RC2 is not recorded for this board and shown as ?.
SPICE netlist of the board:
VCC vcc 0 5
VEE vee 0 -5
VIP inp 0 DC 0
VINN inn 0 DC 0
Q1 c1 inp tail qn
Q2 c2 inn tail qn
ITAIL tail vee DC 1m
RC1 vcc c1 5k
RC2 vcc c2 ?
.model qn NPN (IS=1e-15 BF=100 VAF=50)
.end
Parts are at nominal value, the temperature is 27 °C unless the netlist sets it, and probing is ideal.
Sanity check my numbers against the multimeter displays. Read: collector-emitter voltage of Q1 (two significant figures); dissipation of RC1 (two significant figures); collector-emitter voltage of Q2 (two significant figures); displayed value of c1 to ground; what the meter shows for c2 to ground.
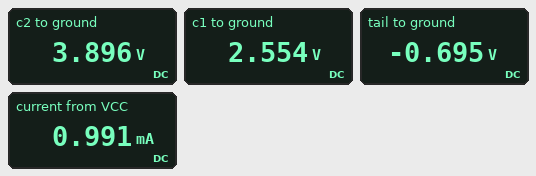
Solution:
3.2 V
1.2 mW
4.6 V
2.554 V
3.896 V
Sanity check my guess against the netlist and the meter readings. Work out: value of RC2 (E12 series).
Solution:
2.2 kΩ
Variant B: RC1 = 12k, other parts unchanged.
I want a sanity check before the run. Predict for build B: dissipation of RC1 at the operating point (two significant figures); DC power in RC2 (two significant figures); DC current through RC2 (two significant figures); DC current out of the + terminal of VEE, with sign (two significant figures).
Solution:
2.6 mW
590 µW
520 µA
-1.0 mA
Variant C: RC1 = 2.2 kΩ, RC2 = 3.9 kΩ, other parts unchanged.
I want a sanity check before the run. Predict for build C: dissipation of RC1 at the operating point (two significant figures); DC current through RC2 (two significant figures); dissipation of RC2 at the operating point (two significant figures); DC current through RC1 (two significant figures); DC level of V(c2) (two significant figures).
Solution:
550 µW
490 µA
940 µW
500 µA
3.1 V
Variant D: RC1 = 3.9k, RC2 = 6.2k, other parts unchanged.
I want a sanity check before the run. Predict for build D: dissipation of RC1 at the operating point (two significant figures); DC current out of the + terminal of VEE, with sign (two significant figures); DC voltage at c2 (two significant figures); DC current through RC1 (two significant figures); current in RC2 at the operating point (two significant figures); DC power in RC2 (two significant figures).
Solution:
980 µW
-1.0 mA
2.0 V
500 µA
490 µA
1.5 mW
